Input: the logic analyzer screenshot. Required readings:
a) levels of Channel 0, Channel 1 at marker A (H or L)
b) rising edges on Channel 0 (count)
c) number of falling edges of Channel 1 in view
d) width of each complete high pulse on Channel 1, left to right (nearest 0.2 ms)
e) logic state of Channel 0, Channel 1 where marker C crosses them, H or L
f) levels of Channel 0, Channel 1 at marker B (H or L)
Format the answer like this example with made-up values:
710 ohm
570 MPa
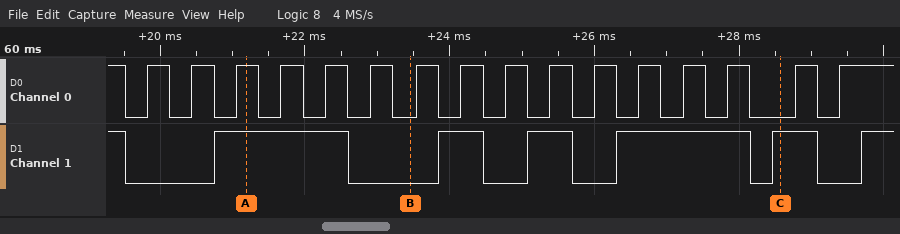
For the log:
Channel 0=H, Channel 1=H
16
6
1.8 ms, 0.6 ms, 0.6 ms, 1.8 ms, 0.6 ms
Channel 0=L, Channel 1=H
Channel 0=L, Channel 1=L
